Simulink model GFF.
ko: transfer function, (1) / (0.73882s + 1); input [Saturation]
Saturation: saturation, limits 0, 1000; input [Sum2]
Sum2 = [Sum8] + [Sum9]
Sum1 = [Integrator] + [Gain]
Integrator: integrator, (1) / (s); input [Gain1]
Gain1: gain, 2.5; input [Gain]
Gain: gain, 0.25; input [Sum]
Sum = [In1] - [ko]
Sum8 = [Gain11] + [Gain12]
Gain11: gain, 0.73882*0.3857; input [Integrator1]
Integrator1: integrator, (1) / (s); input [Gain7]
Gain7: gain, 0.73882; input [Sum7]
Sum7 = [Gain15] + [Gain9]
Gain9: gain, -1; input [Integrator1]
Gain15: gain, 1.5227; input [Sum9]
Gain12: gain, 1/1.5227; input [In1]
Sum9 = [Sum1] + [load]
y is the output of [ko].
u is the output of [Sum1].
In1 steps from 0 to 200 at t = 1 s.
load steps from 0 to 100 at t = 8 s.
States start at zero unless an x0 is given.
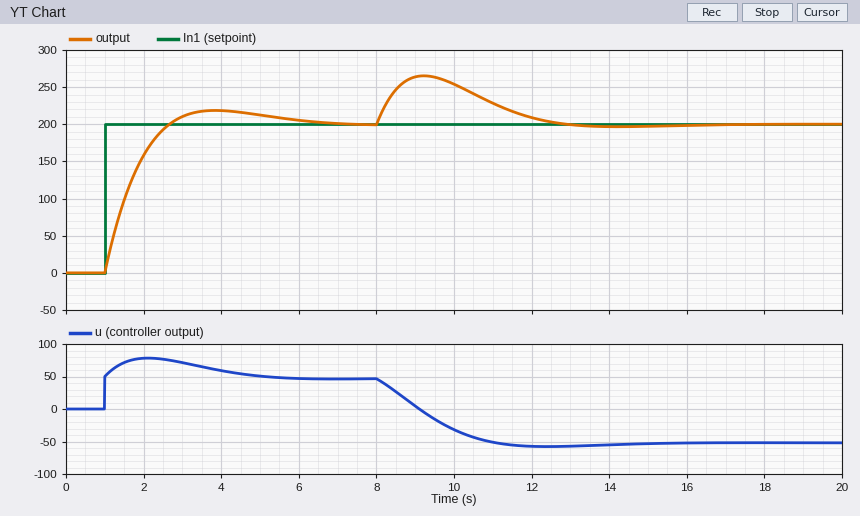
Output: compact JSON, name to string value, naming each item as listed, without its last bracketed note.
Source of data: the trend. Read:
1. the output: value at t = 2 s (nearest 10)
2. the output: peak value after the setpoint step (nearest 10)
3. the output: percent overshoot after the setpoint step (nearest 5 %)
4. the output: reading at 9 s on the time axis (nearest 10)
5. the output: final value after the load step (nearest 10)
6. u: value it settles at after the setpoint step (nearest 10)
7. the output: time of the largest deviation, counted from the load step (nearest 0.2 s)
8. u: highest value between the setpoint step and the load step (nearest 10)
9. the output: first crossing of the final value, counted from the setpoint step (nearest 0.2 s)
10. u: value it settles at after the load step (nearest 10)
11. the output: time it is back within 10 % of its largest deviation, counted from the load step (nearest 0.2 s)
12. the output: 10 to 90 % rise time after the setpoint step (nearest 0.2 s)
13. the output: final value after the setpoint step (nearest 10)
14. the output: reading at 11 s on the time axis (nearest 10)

{"the output: value at t = 2 s": "160", "the output: peak value after the setpoint step": "220", "the output: percent overshoot after the setpoint step": "10 %", "the output: reading at 9 s on the time axis": "260", "the output: final value after the load step": "200", "u: value it settles at after the setpoint step": "50", "the output: time of the largest deviation, counted from the load step": "1.2 s", "u: highest value between the setpoint step and the load step": "80", "the output: first crossing of the final value, counted from the setpoint step": "1.6 s", "u: value it settles at after the load step": "-50", "the output: time it is back within 10 % of its largest deviation, counted from the load step": "4.2 s", "the output: 10 to 90 % rise time after the setpoint step": "1.2 s", "the output: final value after the setpoint step": "200", "the output: reading at 11 s on the time axis": "230"}
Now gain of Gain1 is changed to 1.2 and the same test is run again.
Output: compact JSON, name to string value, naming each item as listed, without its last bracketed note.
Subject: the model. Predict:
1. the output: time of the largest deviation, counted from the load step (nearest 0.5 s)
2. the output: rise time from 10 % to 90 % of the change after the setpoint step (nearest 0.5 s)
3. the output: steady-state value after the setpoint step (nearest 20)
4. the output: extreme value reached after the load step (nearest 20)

{"the output: time of the largest deviation, counted from the load step": "1.5 s", "the output: rise time from 10 % to 90 % of the change after the setpoint step": "2.0 s", "the output: steady-state value after the setpoint step": "200", "the output: extreme value reached after the load step": "280"}
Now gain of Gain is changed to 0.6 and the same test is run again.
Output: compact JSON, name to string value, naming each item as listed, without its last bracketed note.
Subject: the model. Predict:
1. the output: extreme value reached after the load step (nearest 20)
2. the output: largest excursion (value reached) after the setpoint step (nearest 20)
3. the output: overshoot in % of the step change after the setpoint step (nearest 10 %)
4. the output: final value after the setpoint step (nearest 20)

{"the output: extreme value reached after the load step": "240", "the output: largest excursion (value reached) after the setpoint step": "240", "the output: overshoot in % of the step change after the setpoint step": "20 %", "the output: final value after the setpoint step": "200"}
